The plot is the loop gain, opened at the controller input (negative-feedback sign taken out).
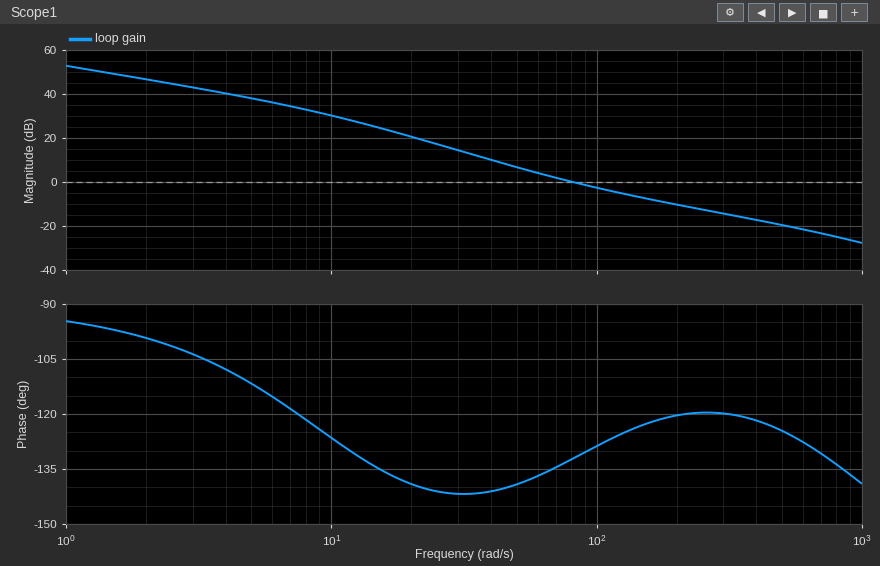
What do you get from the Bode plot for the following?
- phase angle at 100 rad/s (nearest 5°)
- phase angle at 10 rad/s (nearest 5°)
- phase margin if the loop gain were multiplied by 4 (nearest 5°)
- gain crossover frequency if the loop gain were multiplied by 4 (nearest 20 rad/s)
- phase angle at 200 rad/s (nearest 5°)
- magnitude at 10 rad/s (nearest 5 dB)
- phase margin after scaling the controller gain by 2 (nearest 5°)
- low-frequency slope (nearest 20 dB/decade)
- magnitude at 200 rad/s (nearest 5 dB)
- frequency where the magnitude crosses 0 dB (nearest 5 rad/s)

-130°
-125°
60°
240 rad/s
-120°
30 dB
55°
-20 dB/decade
-10 dB
80 rad/s
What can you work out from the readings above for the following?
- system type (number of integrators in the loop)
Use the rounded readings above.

1
